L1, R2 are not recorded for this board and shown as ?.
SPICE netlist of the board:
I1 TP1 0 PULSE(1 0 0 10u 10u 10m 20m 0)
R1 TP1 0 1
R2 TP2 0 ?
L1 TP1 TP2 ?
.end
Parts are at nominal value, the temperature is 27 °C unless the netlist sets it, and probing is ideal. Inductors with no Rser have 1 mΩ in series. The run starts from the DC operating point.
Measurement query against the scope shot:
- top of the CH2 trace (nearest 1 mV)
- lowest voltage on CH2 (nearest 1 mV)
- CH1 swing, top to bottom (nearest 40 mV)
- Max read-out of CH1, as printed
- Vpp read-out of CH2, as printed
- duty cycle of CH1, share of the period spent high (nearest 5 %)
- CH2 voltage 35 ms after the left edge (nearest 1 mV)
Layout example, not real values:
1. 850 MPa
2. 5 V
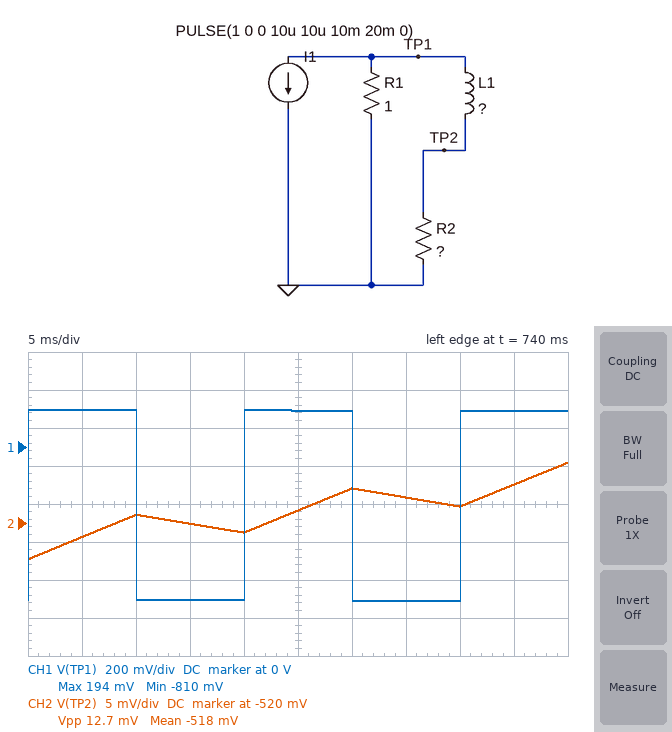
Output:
1. -512 mV
2. -525 mV
3. 1.00 V
4. 194 mV
5. 12.7 mV
6. 50 %
7. -517 mV
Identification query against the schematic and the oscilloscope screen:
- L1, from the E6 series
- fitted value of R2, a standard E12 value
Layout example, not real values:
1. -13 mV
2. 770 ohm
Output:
1. 3.3 H
2. 2.7 Ω
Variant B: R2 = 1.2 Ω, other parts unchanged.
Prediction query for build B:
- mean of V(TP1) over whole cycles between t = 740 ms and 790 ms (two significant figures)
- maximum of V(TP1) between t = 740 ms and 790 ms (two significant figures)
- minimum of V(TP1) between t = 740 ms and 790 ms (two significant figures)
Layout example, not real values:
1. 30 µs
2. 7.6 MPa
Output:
1. -140 mV
2. 370 mV
3. -640 mV
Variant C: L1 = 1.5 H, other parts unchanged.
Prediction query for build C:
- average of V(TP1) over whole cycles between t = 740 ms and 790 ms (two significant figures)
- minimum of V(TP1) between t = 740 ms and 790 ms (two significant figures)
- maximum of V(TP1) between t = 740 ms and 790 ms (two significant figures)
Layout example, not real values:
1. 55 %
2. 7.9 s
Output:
1. -340 mV
2. -850 mV
3. 160 mV
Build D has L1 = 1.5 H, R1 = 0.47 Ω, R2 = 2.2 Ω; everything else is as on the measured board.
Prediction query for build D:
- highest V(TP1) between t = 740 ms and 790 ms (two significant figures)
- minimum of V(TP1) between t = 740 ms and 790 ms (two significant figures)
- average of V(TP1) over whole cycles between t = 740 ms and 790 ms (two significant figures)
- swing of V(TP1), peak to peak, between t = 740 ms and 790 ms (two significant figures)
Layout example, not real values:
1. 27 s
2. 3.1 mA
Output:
1. 53 mV
2. -420 mV
3. -180 mV
4. 470 mV
